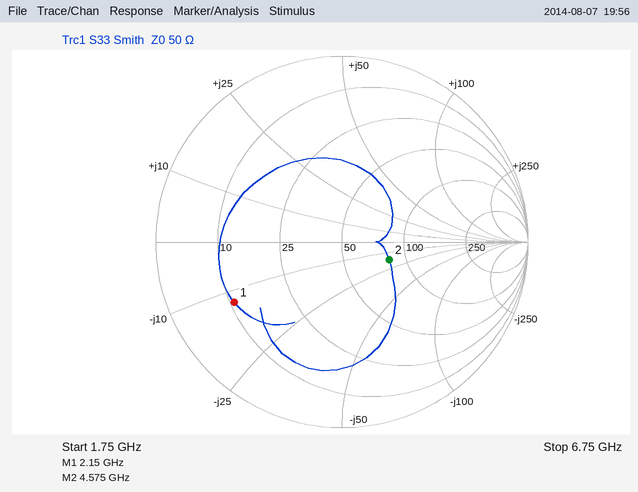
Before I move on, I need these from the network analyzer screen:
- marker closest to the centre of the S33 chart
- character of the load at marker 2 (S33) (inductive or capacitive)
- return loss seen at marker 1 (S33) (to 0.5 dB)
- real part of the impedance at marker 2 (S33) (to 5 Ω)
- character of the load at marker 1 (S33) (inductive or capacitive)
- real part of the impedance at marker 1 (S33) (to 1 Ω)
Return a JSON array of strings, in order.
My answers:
["marker 2", "capacitive", "3.5 dB", "80 Ω", "capacitive", "11 Ω"]
